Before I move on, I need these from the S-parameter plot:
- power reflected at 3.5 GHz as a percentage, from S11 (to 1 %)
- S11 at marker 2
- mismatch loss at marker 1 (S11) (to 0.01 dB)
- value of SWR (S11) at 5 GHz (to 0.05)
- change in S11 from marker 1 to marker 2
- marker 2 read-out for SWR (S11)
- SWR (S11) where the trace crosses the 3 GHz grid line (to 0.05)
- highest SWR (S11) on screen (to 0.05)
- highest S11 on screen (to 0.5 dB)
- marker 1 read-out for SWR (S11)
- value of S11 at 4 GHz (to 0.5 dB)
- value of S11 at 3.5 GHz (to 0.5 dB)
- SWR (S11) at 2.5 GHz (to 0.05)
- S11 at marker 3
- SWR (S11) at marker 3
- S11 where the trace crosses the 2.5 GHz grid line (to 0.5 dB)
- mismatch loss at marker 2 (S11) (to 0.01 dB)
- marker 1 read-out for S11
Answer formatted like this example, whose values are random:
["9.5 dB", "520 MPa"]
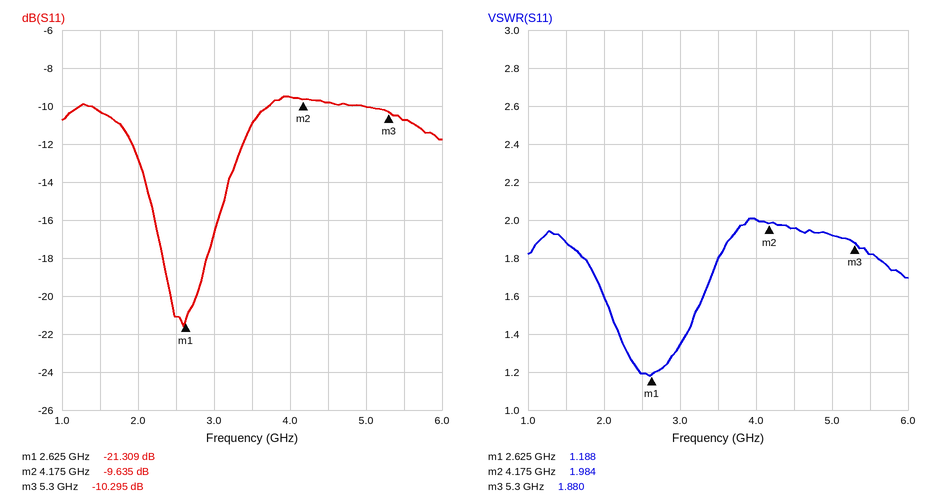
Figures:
["8 %", "-9.635 dB", "0.03 dB", "1.90", "11.674 dB", "1.984", "1.35", "2.00", "-9.5 dB", "1.188", "-9.5 dB", "-11.0 dB", "1.20", "-10.295 dB", "1.880", "-21.0 dB", "0.50 dB", "-21.309 dB"]
